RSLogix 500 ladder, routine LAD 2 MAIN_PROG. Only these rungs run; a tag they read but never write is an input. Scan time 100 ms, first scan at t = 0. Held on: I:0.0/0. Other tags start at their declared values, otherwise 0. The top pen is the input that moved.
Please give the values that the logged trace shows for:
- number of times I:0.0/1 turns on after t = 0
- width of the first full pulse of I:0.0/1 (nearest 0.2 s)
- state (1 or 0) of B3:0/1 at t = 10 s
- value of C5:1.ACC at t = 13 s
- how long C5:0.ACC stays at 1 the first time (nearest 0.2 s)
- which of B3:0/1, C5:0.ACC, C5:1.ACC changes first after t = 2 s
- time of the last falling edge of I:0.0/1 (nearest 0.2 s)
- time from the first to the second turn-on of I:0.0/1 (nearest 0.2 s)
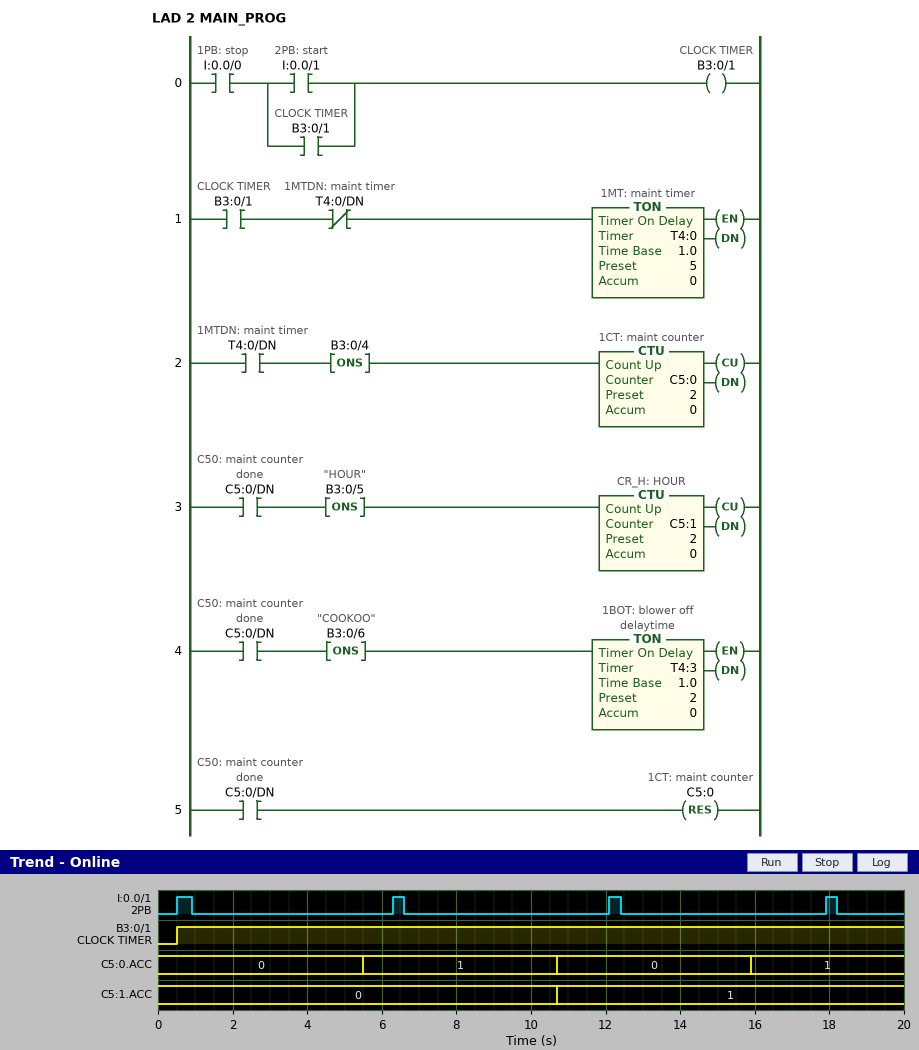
4
0.4 s
1
1
5.2 s
C5:0.ACC
18.2 s
5.8 s
